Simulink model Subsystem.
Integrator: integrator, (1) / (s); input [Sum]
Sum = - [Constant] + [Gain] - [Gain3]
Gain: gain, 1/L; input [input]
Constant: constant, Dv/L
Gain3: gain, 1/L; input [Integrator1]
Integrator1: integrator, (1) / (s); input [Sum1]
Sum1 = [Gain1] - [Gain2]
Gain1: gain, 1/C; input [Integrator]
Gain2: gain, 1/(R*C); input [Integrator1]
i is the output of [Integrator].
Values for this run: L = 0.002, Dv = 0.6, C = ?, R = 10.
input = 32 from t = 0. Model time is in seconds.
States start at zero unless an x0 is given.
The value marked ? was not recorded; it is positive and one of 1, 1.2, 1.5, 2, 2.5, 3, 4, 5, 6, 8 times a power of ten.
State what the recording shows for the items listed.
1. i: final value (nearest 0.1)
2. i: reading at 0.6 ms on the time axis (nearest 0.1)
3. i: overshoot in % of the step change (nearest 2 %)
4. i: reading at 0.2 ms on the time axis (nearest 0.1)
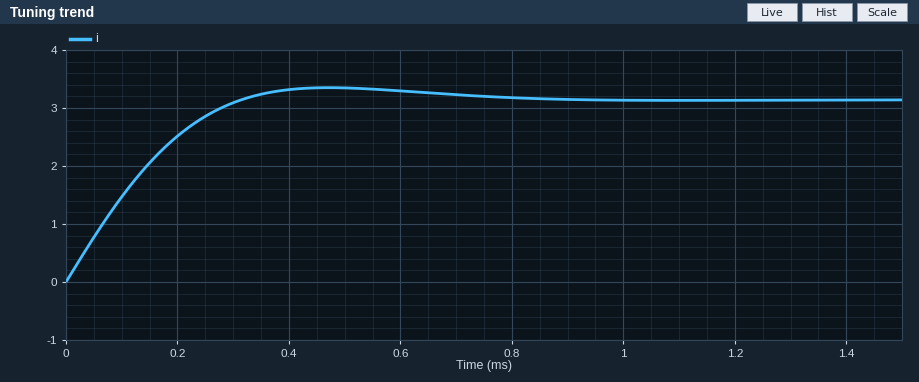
3.1
3.3
6 %
2.5
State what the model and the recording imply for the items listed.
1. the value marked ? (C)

1e-05
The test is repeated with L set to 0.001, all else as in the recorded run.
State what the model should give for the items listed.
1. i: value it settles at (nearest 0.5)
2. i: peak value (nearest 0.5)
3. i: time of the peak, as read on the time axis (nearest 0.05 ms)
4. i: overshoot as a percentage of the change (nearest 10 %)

3.0
4.0
0.25 ms
30 %
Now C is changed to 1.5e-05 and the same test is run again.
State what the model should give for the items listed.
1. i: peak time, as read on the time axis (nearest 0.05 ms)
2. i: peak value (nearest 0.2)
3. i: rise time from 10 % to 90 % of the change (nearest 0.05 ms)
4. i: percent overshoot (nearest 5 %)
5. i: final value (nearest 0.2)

0.45 ms
3.8
0.20 ms
20 %
3.2
